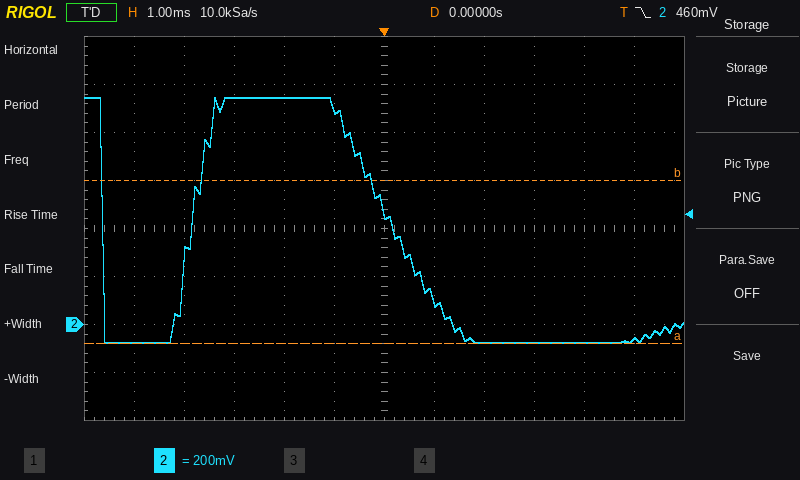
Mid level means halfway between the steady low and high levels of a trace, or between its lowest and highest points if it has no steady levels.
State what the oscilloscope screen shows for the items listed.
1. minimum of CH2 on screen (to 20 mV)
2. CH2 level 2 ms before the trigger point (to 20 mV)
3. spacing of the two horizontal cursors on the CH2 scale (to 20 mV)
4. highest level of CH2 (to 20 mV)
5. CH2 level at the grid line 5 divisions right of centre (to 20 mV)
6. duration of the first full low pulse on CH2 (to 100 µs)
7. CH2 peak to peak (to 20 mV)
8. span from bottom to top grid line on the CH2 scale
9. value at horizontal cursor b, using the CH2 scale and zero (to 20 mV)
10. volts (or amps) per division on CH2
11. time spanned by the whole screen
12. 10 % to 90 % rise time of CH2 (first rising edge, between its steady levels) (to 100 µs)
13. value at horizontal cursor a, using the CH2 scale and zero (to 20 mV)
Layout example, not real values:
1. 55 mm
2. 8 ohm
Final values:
1. -80 mV
2. 940 mV
3. 680 mV
4. 940 mV
5. -60 mV
6. 1.8 ms
7. 1.02 V
8. 1.6 V
9. 600 mV
10. 200 mV
11. 12 ms
12. 800 µs
13. -80 mV
